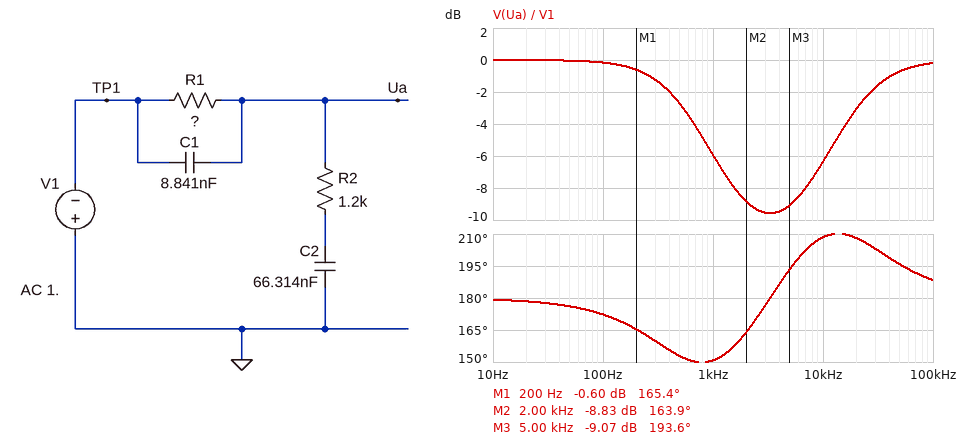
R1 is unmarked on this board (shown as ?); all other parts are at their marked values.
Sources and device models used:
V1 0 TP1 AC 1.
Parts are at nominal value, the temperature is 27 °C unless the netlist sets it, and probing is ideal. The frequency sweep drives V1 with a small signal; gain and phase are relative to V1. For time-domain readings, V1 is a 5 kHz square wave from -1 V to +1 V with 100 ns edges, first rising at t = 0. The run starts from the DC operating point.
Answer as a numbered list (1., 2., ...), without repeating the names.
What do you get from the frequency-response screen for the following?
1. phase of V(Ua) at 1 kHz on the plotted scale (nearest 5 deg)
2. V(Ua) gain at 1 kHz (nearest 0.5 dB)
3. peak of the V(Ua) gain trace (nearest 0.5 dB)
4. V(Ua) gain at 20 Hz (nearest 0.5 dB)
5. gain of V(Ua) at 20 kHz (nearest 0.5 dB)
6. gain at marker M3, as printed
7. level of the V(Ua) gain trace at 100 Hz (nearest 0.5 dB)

1. 150 deg
2. -6.0 dB
3. 0 dB
4. 0 dB
5. -3.0 dB
6. -9.07 dB
7. 0 dB
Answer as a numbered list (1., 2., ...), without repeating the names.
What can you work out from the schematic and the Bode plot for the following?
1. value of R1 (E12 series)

1. 3.3 kΩ
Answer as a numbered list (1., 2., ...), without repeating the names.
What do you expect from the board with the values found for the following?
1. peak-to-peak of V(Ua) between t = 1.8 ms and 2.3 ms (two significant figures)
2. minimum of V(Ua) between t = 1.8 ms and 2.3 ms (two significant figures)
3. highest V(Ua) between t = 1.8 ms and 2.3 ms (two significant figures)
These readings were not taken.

1. 3.2 V
2. -1.6 V
3. 1.6 V
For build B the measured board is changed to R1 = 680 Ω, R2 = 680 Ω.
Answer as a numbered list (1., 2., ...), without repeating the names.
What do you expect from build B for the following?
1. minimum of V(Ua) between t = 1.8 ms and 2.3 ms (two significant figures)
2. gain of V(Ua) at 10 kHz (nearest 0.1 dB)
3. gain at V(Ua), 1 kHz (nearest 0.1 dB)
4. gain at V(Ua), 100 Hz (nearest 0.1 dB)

1. -1.2 V
2. -5.5 dB
3. -0.9 dB
4. 0 dB
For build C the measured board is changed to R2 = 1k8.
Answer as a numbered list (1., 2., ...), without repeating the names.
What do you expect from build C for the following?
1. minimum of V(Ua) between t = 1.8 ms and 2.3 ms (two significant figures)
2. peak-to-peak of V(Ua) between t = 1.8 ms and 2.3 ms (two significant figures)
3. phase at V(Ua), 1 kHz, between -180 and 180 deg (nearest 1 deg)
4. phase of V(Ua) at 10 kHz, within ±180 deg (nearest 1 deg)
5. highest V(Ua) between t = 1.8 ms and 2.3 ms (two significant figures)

1. -1.5 V
2. 3.1 V
3. 158 deg
4. -155 deg
5. 1.5 V
